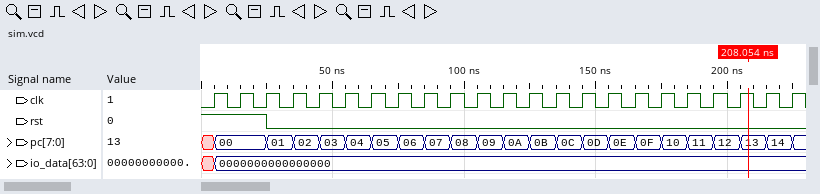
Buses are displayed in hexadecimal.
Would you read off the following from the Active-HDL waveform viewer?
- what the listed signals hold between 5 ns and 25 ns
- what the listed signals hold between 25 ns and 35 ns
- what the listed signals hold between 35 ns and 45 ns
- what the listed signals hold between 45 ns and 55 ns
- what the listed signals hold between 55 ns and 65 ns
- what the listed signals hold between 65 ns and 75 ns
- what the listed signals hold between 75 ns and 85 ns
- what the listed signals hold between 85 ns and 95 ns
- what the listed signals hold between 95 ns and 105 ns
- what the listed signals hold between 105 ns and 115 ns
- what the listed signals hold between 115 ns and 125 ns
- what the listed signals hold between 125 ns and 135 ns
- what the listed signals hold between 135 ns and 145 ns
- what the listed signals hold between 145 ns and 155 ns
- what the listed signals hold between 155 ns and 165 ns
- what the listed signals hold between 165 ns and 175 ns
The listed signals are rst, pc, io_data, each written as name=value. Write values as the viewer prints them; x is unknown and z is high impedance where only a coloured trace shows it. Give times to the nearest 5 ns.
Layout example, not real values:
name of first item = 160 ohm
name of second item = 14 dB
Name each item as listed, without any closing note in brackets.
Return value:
what the listed signals hold between 5 ns and 25 ns = rst=1, pc=00, io_data=0000000000000000
what the listed signals hold between 25 ns and 35 ns = rst=0, pc=01, io_data=0000000000000000
what the listed signals hold between 35 ns and 45 ns = rst=0, pc=02, io_data=0000000000000000
what the listed signals hold between 45 ns and 55 ns = rst=0, pc=03, io_data=0000000000000000
what the listed signals hold between 55 ns and 65 ns = rst=0, pc=04, io_data=0000000000000000
what the listed signals hold between 65 ns and 75 ns = rst=0, pc=05, io_data=0000000000000000
what the listed signals hold between 75 ns and 85 ns = rst=0, pc=06, io_data=0000000000000000
what the listed signals hold between 85 ns and 95 ns = rst=0, pc=07, io_data=0000000000000000
what the listed signals hold between 95 ns and 105 ns = rst=0, pc=08, io_data=0000000000000000
what the listed signals hold between 105 ns and 115 ns = rst=0, pc=09, io_data=0000000000000000
what the listed signals hold between 115 ns and 125 ns = rst=0, pc=0A, io_data=0000000000000000
what the listed signals hold between 125 ns and 135 ns = rst=0, pc=0B, io_data=0000000000000000
what the listed signals hold between 135 ns and 145 ns = rst=0, pc=0C, io_data=0000000000000000
what the listed signals hold between 145 ns and 155 ns = rst=0, pc=0D, io_data=0000000000000000
what the listed signals hold between 155 ns and 165 ns = rst=0, pc=0E, io_data=0000000000000000
what the listed signals hold between 165 ns and 175 ns = rst=0, pc=0F, io_data=0000000000000000
